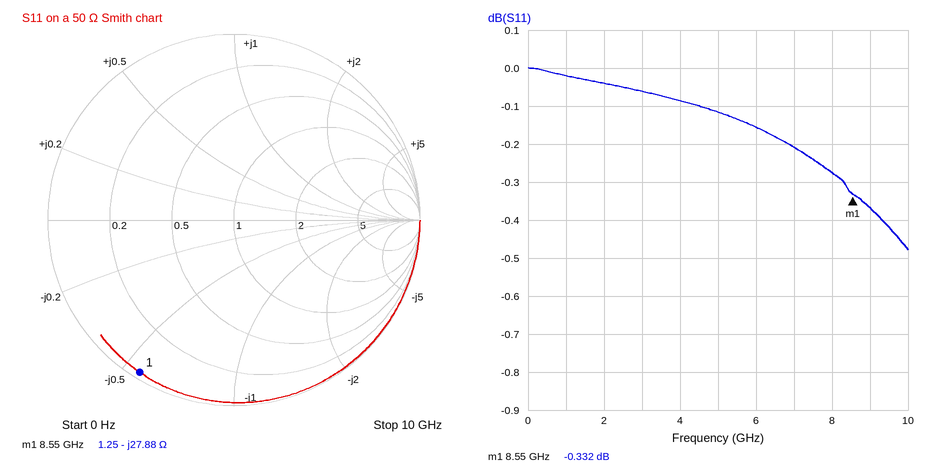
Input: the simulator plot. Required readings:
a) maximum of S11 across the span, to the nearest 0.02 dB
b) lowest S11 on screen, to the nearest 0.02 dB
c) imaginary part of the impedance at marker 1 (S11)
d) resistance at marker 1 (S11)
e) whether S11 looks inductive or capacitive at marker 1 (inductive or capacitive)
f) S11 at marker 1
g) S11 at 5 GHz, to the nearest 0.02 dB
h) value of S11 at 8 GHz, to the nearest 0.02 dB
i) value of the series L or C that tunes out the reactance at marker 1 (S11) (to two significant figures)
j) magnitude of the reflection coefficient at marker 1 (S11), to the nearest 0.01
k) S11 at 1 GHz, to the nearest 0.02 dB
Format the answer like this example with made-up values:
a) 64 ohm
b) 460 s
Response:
a) 0.00 dB
b) -0.48 dB
c) -27.88 Ω
d) 1.25 Ω
e) capacitive
f) -0.332 dB
g) -0.12 dB
h) -0.28 dB
i) 520 pH
j) 0.96
k) -0.02 dB
